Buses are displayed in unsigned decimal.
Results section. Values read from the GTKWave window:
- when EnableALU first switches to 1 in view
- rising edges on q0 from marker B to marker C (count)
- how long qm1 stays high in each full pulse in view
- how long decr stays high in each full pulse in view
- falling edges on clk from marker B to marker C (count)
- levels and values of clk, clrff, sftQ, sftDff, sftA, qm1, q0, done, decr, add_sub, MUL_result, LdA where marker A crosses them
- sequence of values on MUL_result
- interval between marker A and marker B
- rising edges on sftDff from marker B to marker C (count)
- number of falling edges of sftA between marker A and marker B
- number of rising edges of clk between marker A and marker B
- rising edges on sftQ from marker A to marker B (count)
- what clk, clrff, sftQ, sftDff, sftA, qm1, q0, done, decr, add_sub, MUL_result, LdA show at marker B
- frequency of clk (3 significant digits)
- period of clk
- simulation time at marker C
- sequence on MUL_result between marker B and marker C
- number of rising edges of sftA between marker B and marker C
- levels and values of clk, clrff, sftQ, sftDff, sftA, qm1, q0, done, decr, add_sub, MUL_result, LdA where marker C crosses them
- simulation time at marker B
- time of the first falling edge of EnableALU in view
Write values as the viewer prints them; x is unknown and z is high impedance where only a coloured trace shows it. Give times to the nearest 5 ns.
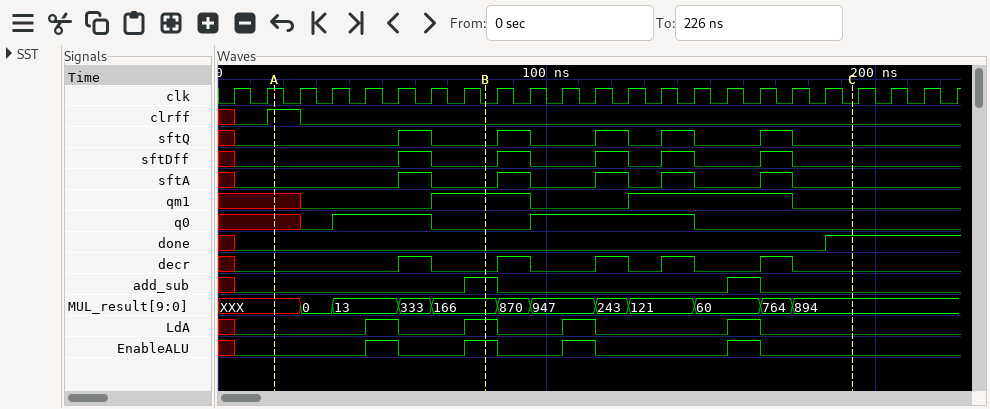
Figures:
45 ns
1
30 ns, 50 ns
10 ns, 10 ns, 10 ns, 10 ns, 10 ns
11
clk=1, clrff=1, sftQ=0, sftDff=0, sftA=0, qm1=x, q0=x, done=0, decr=0, add_sub=0, MUL_result=XXX, LdA=0
XXX, 0, 13, 333, 166, 870, 947, 243, 121, 60, 764, 894
65 ns
4
1
6
1
clk=0, clrff=0, sftQ=0, sftDff=0, sftA=0, qm1=1, q0=0, done=0, decr=0, add_sub=1, MUL_result=166, LdA=1
100 MHz
10 ns
195 ns
166, 870, 947, 243, 121, 60, 764, 894
4
clk=0, clrff=0, sftQ=0, sftDff=0, sftA=0, qm1=0, q0=0, done=1, decr=0, add_sub=0, MUL_result=894, LdA=0
80 ns
55 ns
